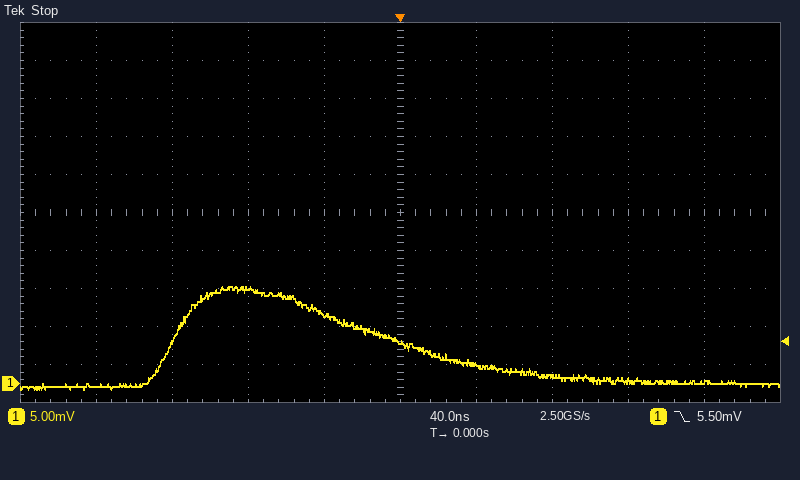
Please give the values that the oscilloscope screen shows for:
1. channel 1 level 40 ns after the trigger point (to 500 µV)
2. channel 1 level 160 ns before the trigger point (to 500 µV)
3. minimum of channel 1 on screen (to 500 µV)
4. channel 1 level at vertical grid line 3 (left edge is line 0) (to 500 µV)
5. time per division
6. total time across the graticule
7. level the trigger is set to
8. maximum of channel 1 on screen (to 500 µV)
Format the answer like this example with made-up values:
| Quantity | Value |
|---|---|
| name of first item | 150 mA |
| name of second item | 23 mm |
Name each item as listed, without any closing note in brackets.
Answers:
| Quantity | Value |
|---|---|
| channel 1 level 40 ns after the trigger point | 2.5 mV |
| channel 1 level 160 ns before the trigger point | -500 µV |
| minimum of channel 1 on screen | -1.0 mV |
| channel 1 level at vertical grid line 3 (left edge is line 0) | 12.5 mV |
| time per division | 40 ns |
| total time across the graticule | 400 ns |
| level the trigger is set to | 5.50 mV |
| maximum of channel 1 on screen | 13.0 mV |
